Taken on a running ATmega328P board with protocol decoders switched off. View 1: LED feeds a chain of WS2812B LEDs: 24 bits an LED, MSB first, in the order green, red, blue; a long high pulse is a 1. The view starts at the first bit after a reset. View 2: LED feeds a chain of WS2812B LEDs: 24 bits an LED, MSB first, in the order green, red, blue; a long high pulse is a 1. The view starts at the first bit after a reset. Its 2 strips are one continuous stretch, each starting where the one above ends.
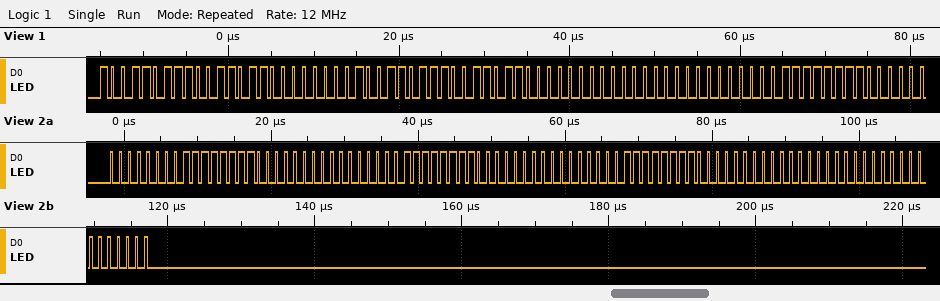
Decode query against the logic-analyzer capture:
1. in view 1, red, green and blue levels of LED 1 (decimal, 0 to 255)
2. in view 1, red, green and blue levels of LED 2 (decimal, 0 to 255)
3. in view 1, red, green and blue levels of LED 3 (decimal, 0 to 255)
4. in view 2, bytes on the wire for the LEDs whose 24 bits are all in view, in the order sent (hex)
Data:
155, 155, 0
155, 155, 0
0, 0, 255
00 FF 00 00 FF 00 00 FF 00 00 00 00
